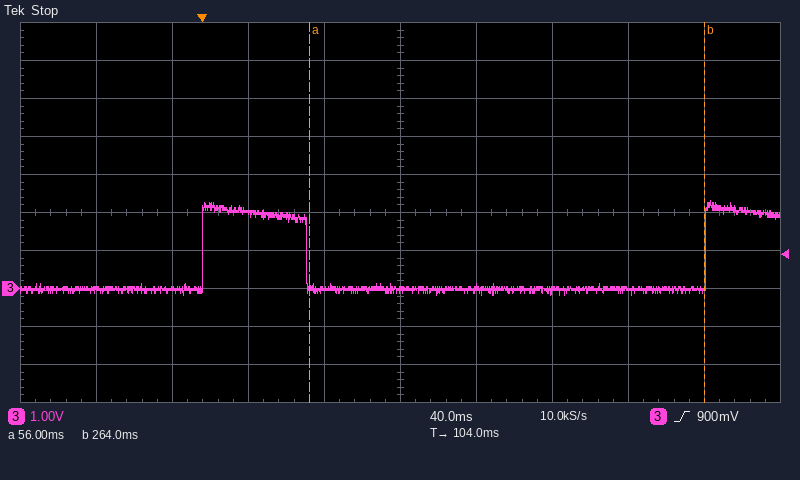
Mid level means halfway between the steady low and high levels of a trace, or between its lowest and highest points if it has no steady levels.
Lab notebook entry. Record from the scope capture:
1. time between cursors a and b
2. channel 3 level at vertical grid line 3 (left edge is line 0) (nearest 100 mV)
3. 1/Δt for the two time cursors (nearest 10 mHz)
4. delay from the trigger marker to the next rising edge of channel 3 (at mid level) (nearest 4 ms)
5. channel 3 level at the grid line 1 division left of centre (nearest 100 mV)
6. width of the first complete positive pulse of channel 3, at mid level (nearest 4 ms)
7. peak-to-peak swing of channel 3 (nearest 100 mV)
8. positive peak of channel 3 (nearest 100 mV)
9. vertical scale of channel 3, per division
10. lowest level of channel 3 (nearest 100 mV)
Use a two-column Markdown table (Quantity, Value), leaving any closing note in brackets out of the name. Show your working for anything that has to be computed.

| Quantity | Value |
|---|---|
| time between cursors a and b | 264 ms − (56 ms) = 208 ms |
| channel 3 level at vertical grid line 3 (left edge is line 0) | 2.0 V |
| 1/Δt for the two time cursors | 1 / 208 ms ≈ 4.81 Hz |
| delay from the trigger marker to the next rising edge of channel 3 (at mid level) | 264 ms |
| channel 3 level at the grid line 1 division left of centre | 0.0 V |
| width of the first complete positive pulse of channel 3, at mid level | 56 ms |
| peak-to-peak swing of channel 3 | 2.3 V − (-200 mV) = 2.5 V |
| positive peak of channel 3 | 2.3 V |
| vertical scale of channel 3, per division | 1 V |
| lowest level of channel 3 | -200 mV |
